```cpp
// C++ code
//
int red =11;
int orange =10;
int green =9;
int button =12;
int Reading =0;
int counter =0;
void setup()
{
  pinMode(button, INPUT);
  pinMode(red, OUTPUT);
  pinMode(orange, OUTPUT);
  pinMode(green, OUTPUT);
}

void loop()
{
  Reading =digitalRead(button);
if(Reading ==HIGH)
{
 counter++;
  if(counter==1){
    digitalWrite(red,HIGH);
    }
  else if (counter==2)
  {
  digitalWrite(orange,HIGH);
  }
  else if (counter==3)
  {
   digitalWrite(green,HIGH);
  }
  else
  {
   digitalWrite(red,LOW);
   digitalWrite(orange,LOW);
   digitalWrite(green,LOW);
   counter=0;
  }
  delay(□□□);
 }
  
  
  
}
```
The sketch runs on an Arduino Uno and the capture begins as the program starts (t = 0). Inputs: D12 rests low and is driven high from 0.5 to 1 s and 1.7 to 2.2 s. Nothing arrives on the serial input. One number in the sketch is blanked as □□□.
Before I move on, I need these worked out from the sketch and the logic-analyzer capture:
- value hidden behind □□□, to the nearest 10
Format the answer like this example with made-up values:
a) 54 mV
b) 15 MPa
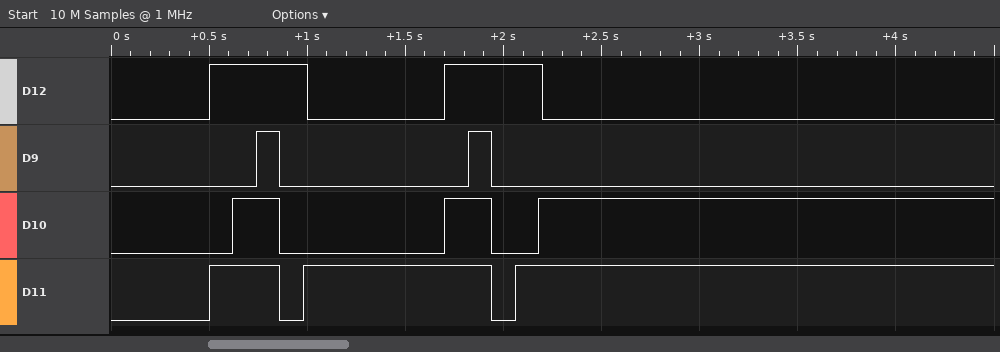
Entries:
a) 120
